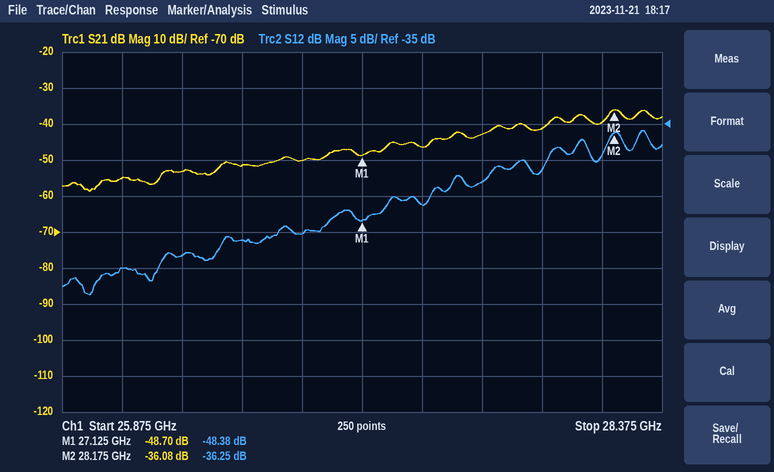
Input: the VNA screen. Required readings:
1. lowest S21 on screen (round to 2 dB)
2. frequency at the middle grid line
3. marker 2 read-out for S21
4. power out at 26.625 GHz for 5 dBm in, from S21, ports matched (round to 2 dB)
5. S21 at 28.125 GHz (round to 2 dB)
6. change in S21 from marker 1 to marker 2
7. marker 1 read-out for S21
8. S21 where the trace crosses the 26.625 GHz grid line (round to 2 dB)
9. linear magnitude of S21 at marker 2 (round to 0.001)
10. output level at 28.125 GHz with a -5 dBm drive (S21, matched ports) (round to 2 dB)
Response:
-58 dB
27.125 GHz
-36.08 dB
-46 dBm
-40 dB
12.62 dB
-48.70 dB
-52 dB
0.016
-44 dBm
